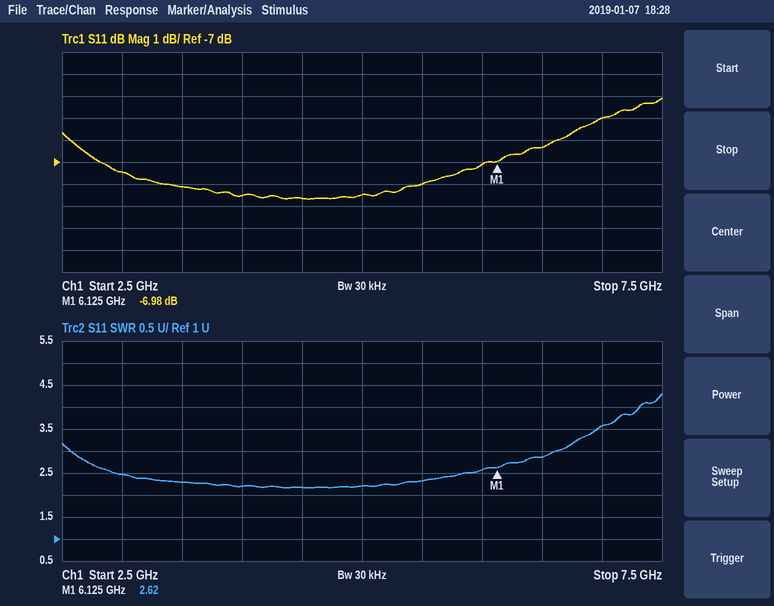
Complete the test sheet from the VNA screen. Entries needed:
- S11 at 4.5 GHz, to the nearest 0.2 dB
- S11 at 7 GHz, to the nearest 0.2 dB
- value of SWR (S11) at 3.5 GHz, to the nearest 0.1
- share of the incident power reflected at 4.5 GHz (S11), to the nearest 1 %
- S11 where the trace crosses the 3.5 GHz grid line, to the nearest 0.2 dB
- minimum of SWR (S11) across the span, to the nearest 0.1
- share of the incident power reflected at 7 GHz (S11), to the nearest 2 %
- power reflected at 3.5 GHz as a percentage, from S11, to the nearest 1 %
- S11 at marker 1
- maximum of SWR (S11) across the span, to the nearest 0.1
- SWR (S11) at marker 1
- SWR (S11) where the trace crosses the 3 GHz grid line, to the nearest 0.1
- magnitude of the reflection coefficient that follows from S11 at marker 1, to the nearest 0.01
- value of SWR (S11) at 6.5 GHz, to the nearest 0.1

-8.6 dB
-5.0 dB
2.3
14 %
-8.2 dB
2.2
32 %
15 %
-6.98 dB
4.3
2.62
2.5
0.45
2.9
